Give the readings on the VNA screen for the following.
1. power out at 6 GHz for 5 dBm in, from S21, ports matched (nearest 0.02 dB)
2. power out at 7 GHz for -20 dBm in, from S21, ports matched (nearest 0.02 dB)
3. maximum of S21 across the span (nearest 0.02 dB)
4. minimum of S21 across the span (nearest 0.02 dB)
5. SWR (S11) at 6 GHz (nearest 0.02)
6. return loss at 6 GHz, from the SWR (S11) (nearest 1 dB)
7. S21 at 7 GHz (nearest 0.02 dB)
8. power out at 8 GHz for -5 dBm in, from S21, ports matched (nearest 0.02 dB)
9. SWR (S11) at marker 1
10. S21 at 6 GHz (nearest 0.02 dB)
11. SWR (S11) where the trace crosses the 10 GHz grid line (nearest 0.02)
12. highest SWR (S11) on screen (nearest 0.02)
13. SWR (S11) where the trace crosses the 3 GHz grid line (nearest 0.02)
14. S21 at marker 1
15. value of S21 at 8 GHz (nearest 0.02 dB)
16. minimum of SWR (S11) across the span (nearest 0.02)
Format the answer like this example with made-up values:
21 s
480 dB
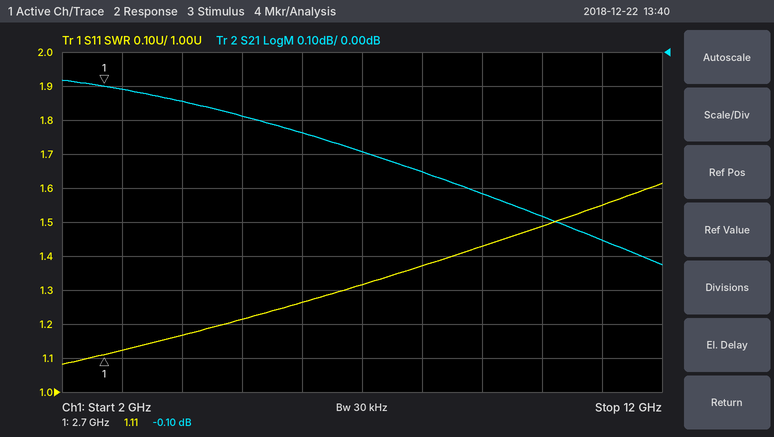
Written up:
4.76 dBm
-20.30 dBm
-0.08 dB
-0.62 dB
1.26
19 dB
-0.30 dB
-5.36 dBm
1.11
-0.24 dB
1.48
1.62
1.12
-0.10 dB
-0.36 dB
1.08
